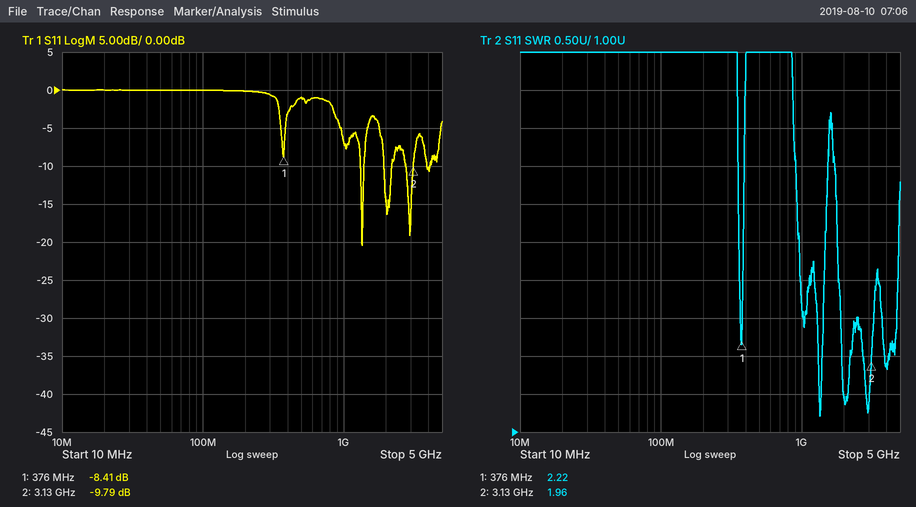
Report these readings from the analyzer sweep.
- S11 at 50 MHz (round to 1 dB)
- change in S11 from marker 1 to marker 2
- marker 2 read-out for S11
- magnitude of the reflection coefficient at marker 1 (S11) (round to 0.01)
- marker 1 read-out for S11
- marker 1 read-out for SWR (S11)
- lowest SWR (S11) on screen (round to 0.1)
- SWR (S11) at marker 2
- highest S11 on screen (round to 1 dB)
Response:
0 dB
-1.38 dB
-9.79 dB
0.38
-8.41 dB
2.22
1.2
1.96
0 dB
